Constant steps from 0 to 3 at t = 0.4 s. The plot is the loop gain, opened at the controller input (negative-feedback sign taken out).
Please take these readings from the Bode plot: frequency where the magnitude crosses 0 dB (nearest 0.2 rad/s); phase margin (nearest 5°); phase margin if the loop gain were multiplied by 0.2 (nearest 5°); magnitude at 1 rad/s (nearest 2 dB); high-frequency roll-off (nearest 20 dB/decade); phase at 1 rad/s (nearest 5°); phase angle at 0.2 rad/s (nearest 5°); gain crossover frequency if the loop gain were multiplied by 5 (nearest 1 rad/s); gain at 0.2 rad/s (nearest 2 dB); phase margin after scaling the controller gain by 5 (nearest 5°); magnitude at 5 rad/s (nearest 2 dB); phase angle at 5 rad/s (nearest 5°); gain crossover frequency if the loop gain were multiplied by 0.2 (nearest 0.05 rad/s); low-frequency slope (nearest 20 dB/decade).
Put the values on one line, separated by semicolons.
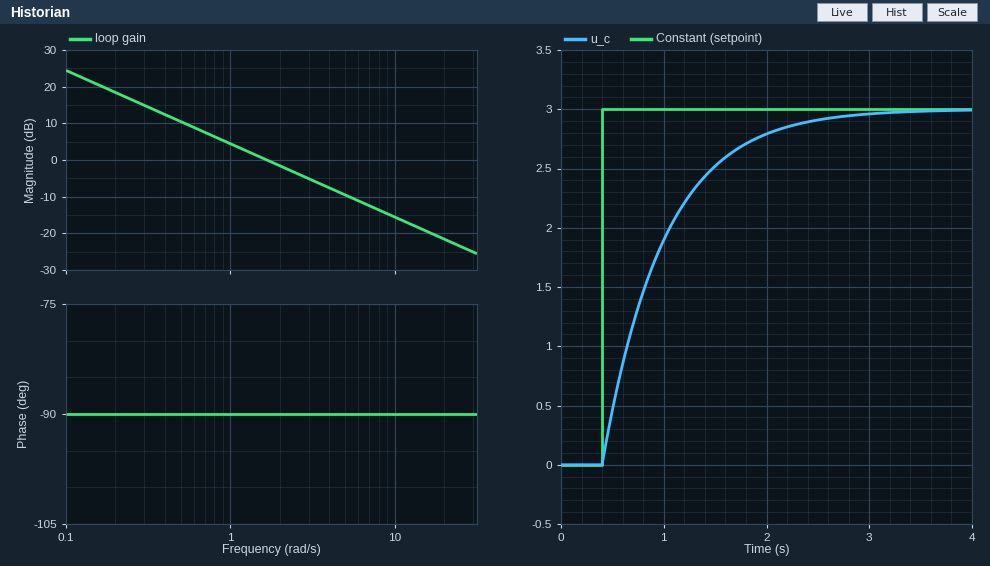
1.6 rad/s; 90°; 90°; 4 dB; -20 dB/decade; -90°; -90°; 8 rad/s; 18 dB; 90°; -10 dB; -90°; 0.35 rad/s; -20 dB/decade
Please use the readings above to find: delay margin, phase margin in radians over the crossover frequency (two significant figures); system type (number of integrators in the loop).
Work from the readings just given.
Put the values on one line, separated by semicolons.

0.98 s; 1
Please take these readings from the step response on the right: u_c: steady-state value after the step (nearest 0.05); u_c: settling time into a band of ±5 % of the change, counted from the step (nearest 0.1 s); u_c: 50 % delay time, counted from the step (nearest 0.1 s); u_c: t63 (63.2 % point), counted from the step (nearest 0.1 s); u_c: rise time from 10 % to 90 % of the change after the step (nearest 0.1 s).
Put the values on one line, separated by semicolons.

3.00; 1.8 s; 0.4 s; 0.6 s; 1.3 s
